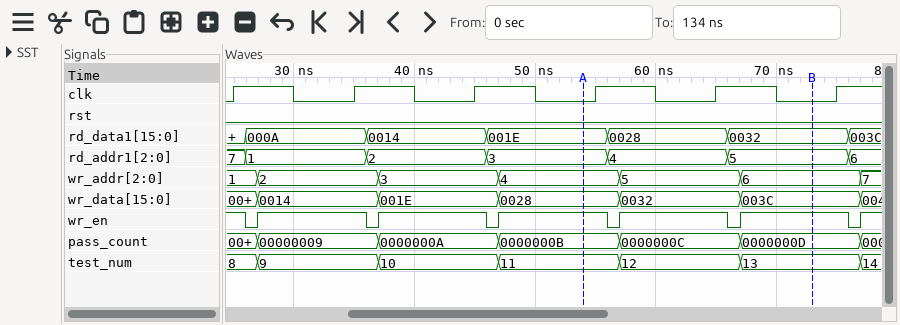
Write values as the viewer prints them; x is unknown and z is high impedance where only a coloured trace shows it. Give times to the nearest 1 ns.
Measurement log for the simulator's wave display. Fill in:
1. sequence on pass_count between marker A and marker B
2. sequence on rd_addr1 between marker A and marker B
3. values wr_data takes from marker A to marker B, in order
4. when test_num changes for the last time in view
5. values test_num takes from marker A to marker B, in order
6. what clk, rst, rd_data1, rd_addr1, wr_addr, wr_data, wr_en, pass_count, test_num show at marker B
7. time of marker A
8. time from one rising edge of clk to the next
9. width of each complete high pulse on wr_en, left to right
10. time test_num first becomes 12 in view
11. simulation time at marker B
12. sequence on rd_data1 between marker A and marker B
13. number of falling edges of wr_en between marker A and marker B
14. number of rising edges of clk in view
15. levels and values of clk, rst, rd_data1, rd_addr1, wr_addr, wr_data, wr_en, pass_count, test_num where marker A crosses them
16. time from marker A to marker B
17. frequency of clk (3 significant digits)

0000000B, 0000000C, 0000000D
3, 4, 5
0028, 0032, 003C
77 ns
11, 12, 13
clk=0, rst=0, rd_data1=0032, rd_addr1=5, wr_addr=6, wr_data=003C, wr_en=1, pass_count=0000000D, test_num=13
54 ns
10 ns
9 ns, 9 ns, 9 ns, 9 ns, 9 ns
57 ns
73 ns
001E, 0028, 0032
2
6
clk=0, rst=0, rd_data1=001E, rd_addr1=3, wr_addr=4, wr_data=0028, wr_en=1, pass_count=0000000B, test_num=11
19 ns
100 MHz
